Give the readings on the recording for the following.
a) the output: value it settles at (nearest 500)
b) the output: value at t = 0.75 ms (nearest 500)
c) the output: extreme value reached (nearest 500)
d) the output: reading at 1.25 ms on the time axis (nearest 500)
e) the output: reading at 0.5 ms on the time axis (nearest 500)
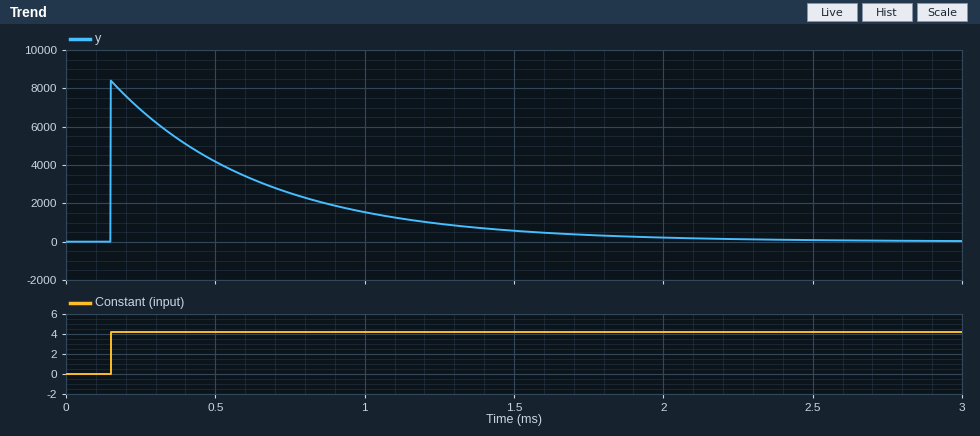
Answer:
0
2500
8500
1000
4000
